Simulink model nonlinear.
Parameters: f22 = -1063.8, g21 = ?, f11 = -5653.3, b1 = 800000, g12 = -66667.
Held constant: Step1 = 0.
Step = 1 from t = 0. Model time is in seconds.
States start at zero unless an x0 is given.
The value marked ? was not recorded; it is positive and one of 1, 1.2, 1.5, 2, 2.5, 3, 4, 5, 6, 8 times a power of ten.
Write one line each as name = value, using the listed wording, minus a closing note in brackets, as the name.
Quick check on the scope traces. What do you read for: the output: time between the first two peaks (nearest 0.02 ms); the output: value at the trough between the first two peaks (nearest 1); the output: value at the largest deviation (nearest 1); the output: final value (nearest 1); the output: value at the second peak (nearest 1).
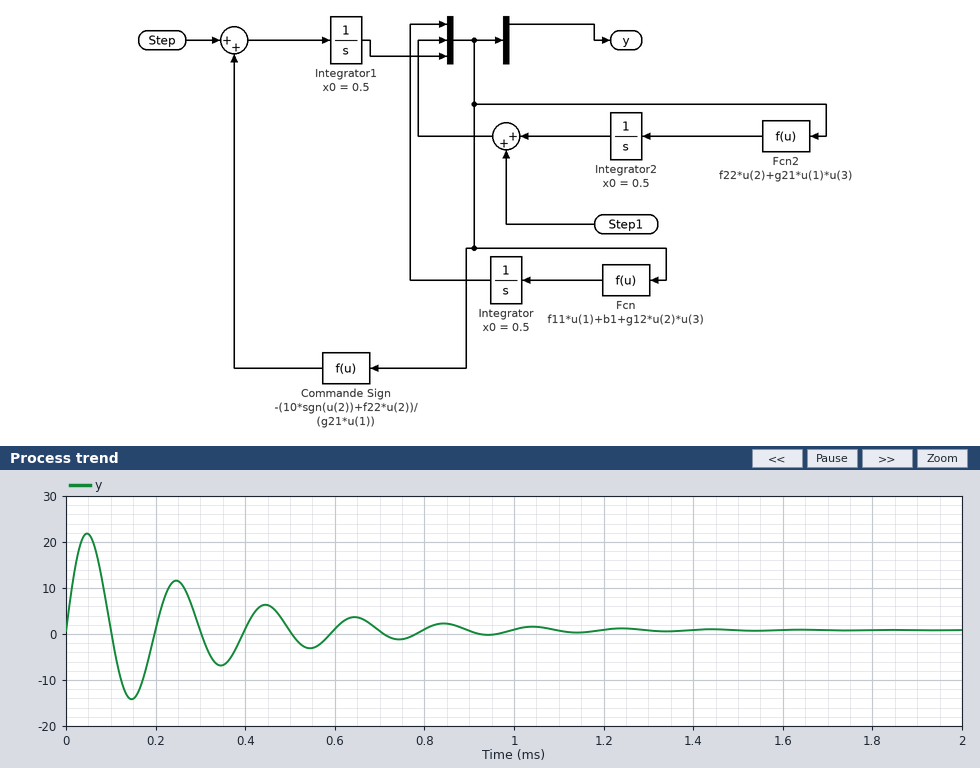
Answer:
the output: time between the first two peaks = 0.20 ms
the output: value at the trough between the first two peaks = -14
the output: value at the largest deviation = 22
the output: final value = 1
the output: value at the second peak = 12
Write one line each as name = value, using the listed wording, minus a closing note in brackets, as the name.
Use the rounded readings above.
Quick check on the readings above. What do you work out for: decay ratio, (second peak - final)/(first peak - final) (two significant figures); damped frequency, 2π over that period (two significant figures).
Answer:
decay ratio, (second peak - final)/(first peak - final) = 0.52
damped frequency, 2π over that period = 31 rad/ms
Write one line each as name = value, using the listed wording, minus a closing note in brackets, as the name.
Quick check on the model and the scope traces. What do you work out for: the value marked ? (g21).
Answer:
the value marked ? = 60000
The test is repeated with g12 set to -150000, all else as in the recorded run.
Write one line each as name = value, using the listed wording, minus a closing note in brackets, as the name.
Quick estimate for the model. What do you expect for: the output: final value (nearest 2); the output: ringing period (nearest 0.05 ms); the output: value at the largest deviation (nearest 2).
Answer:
the output: final value = 0
the output: ringing period = 0.15 ms
the output: value at the largest deviation = 14
